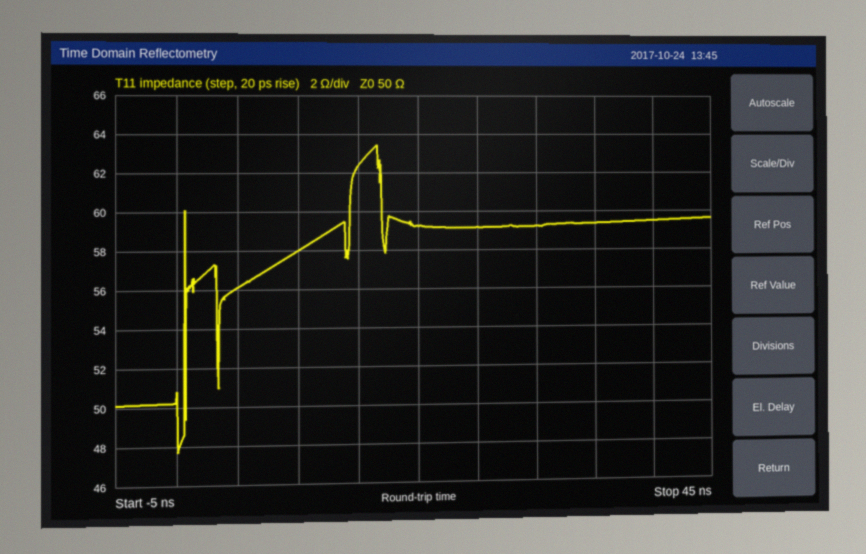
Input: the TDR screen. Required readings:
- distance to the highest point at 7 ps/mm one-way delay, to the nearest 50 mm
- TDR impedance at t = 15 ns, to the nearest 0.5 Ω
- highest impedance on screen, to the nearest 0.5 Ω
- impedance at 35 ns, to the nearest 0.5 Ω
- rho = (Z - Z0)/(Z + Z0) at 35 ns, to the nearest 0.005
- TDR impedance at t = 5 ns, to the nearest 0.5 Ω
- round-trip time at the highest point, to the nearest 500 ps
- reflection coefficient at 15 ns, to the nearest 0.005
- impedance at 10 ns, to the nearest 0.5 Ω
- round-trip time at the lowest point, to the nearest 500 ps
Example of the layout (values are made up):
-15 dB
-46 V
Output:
1.20 m
62.5 Ω
63.5 Ω
59.5 Ω
+0.085
56.0 Ω
16.5 ns
+0.110
58.0 Ω
0.0 ns
